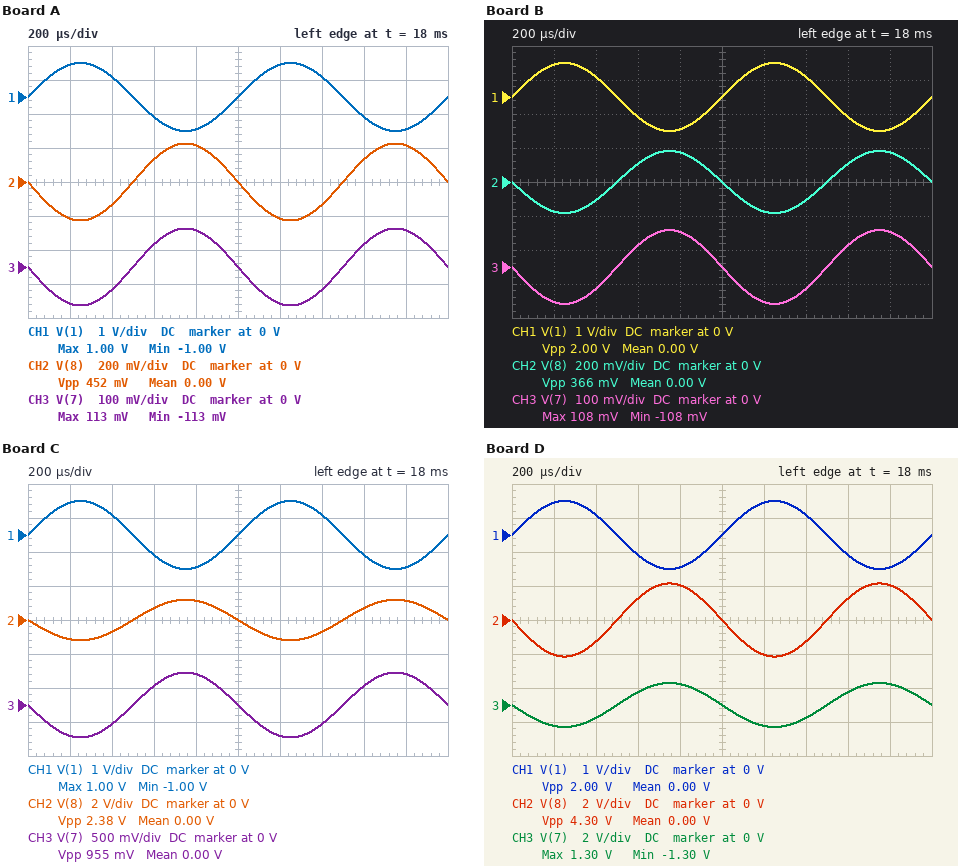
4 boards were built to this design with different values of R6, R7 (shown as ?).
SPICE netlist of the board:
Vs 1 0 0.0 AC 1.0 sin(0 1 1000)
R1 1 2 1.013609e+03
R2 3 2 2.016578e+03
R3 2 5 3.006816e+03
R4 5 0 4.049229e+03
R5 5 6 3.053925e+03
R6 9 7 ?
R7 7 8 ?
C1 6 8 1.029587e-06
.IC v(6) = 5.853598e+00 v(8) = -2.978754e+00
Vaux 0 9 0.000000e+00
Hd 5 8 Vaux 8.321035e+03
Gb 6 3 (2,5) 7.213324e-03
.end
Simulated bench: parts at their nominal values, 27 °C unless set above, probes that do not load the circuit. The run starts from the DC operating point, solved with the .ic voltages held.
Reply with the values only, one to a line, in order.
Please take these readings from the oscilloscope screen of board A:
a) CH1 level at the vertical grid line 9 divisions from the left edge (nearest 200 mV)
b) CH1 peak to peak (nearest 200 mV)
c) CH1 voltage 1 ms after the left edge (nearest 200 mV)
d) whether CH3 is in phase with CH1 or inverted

-1.0 V
2.0 V
0 V
inverted
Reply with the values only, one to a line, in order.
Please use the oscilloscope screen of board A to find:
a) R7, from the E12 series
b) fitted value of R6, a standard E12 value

820 Ω
820 Ω
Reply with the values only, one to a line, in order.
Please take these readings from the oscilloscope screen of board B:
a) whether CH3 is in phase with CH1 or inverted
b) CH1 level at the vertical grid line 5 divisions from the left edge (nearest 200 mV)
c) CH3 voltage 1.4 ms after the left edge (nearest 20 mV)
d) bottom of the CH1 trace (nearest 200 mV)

inverted
0 V
-60 mV
-1.0 V
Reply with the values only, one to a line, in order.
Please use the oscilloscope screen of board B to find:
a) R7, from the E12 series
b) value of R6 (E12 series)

560 Ω
820 Ω
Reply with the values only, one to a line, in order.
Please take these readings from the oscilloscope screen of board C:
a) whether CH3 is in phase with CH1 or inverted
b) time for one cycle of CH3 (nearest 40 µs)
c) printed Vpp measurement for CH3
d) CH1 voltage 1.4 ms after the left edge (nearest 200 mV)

inverted
1.00 ms
955 mV
600 mV
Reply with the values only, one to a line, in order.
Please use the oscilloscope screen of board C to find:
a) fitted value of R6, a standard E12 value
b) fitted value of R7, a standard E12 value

1.8 kΩ
2.7 kΩ
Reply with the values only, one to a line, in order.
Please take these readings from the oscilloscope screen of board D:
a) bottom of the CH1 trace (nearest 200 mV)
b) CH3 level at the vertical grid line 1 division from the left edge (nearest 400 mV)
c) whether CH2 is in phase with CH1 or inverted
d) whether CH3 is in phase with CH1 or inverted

-1.0 V
-1.2 V
inverted
inverted
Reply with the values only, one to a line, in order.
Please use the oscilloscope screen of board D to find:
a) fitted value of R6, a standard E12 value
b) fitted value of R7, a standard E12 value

3.3 kΩ
2.2 kΩ
